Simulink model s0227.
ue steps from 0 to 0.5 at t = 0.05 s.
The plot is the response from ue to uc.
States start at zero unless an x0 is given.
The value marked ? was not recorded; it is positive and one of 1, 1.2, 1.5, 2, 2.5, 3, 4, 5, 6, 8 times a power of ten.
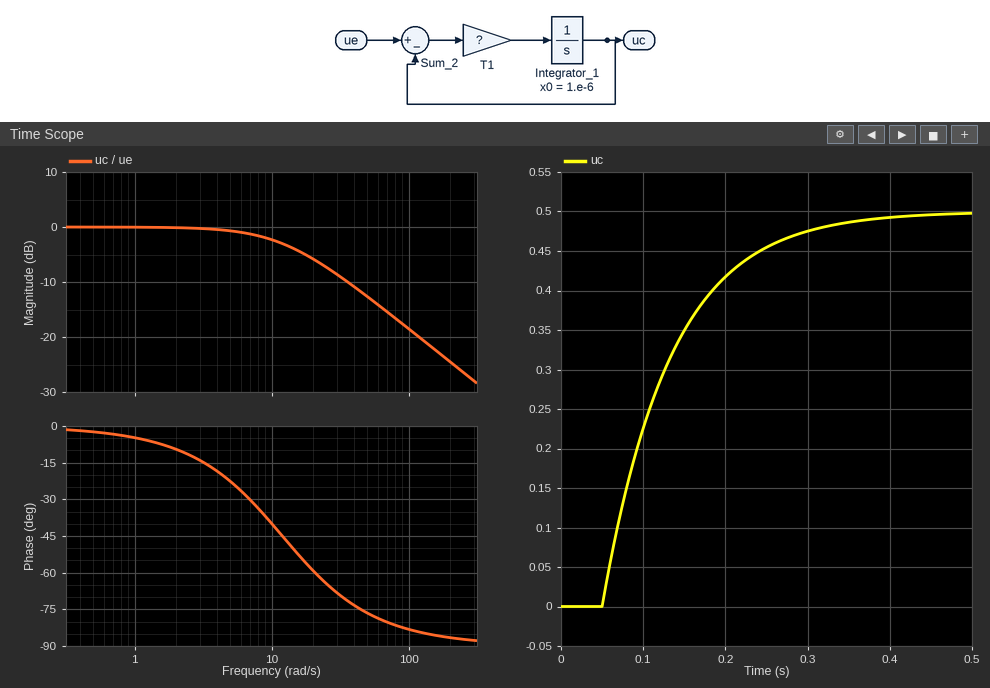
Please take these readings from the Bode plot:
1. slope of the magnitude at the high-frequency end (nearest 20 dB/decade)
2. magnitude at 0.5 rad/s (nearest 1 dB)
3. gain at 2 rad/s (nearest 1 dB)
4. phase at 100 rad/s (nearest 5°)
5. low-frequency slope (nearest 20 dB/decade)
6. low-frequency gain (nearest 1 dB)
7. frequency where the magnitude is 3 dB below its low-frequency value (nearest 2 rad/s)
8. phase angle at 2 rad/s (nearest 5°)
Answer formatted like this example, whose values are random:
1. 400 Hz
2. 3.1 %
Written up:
1. -20 dB/decade
2. 0 dB
3. 0 dB
4. -85°
5. 0 dB/decade
6. 0 dB
7. 12 rad/s
8. -10°
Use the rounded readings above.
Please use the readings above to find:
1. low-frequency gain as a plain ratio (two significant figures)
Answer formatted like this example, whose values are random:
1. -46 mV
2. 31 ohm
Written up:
1. 1.0
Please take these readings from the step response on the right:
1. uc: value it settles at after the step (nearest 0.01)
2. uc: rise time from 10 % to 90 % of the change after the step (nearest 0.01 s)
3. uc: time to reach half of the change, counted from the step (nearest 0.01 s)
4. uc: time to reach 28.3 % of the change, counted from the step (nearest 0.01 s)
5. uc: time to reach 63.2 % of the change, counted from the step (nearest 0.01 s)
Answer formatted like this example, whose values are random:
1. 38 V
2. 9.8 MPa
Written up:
1. 0.50
2. 0.18 s
3. 0.06 s
4. 0.03 s
5. 0.08 s
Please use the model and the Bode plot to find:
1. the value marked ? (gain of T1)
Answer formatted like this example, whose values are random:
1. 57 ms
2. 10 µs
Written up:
1. 12
